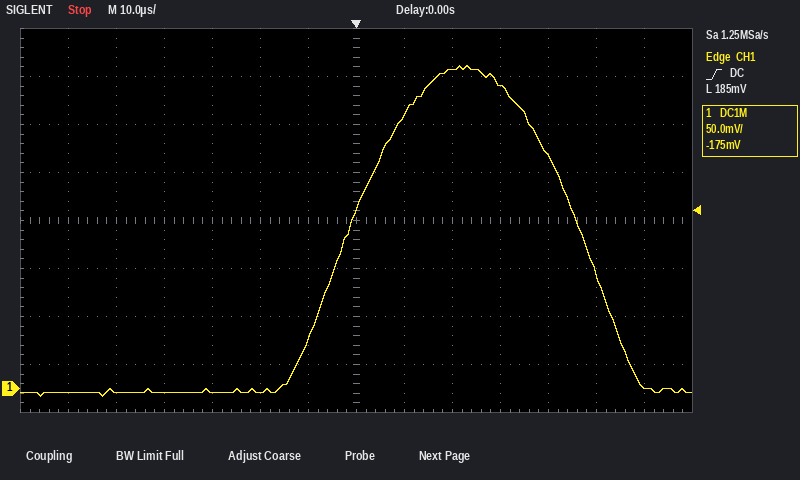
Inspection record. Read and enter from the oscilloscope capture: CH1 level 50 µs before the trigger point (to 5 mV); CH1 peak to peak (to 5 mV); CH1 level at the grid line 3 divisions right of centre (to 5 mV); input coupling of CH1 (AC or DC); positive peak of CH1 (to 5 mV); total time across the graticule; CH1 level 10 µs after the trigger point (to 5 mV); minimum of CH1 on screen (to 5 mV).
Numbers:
-5 mV
345 mV
315 mV
DC
335 mV
140 µs
285 mV
-10 mV
